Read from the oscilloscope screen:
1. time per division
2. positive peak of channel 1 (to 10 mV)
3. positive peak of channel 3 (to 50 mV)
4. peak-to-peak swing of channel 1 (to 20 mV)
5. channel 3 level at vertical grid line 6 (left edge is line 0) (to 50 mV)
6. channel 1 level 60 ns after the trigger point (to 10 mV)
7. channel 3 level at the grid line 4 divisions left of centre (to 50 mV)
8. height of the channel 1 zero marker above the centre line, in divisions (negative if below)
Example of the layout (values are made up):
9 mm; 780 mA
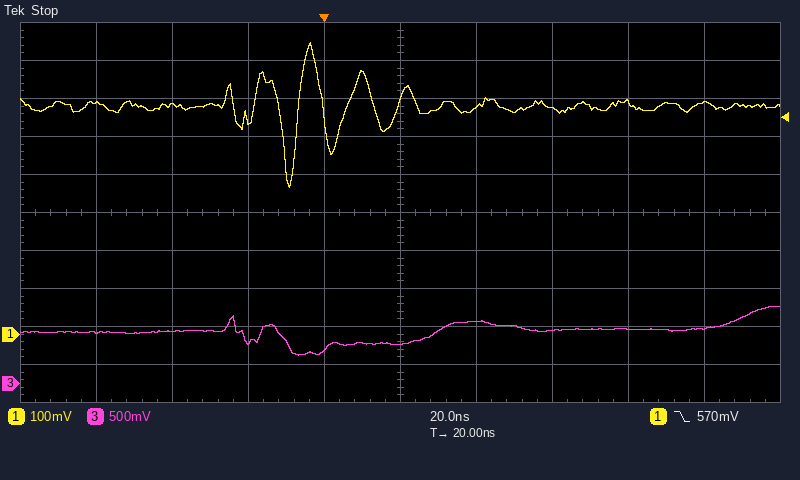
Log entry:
20 ns; 770 mV; 1.00 V; 380 mV; 800 mV; 590 mV; 650 mV; -3.2 div
